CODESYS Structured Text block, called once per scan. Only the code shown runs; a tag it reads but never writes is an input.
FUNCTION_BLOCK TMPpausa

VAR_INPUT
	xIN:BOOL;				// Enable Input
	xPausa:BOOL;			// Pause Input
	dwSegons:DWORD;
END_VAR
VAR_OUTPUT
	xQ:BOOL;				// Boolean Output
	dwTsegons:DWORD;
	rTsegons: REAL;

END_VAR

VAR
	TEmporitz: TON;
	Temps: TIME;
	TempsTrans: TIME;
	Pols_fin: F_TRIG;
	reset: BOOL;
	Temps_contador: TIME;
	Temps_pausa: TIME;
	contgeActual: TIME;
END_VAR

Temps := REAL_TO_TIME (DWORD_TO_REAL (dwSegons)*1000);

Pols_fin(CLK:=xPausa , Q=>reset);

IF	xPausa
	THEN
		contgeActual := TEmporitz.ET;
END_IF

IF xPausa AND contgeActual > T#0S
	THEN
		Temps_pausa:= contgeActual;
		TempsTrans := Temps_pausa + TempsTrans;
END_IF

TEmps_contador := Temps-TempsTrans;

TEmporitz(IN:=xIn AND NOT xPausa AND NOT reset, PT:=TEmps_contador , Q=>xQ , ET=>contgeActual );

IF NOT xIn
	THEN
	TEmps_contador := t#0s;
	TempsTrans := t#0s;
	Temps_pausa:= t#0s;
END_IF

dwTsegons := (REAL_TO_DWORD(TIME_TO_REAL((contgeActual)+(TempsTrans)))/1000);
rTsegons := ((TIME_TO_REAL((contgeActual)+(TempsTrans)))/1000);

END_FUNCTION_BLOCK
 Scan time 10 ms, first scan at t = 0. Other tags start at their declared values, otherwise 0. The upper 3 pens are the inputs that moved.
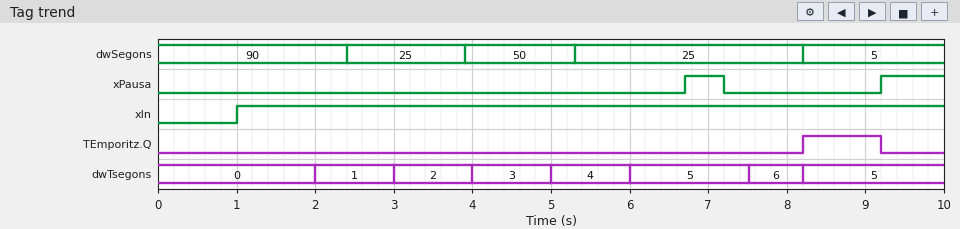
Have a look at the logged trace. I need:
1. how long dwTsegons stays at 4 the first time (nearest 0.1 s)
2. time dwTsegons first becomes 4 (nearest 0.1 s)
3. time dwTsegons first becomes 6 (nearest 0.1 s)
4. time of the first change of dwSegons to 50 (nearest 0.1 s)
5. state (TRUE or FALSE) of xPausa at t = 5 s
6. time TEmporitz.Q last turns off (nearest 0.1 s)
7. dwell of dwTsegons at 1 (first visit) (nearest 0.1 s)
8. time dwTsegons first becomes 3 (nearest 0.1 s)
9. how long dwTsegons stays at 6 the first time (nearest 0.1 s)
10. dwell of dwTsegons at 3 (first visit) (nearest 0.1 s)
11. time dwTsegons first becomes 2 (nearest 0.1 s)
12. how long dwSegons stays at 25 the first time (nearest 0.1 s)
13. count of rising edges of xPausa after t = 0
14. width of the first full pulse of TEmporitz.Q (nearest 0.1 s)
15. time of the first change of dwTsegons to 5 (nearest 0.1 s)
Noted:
1.0 s
5.0 s
7.5 s
3.9 s
FALSE
9.2 s
1.0 s
4.0 s
0.7 s
1.0 s
3.0 s
1.5 s
2
1.0 s
6.0 s
